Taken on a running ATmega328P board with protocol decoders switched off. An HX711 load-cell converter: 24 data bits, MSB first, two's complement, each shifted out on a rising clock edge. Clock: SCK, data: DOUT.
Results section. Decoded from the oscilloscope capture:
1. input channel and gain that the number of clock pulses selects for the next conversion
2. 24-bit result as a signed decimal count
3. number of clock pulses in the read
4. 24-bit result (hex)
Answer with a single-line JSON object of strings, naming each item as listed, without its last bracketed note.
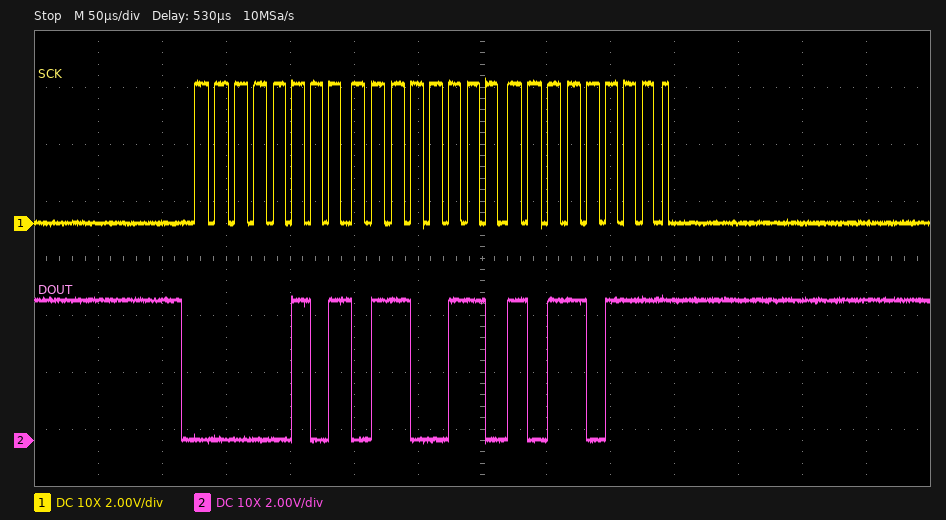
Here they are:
{"input channel and gain that the number of clock pulses selects for the next conversion": "channel A, gain 128", "24-bit result as a signed decimal count": "353975", "number of clock pulses in the read": "25", "24-bit result": "0x0566B7"}
